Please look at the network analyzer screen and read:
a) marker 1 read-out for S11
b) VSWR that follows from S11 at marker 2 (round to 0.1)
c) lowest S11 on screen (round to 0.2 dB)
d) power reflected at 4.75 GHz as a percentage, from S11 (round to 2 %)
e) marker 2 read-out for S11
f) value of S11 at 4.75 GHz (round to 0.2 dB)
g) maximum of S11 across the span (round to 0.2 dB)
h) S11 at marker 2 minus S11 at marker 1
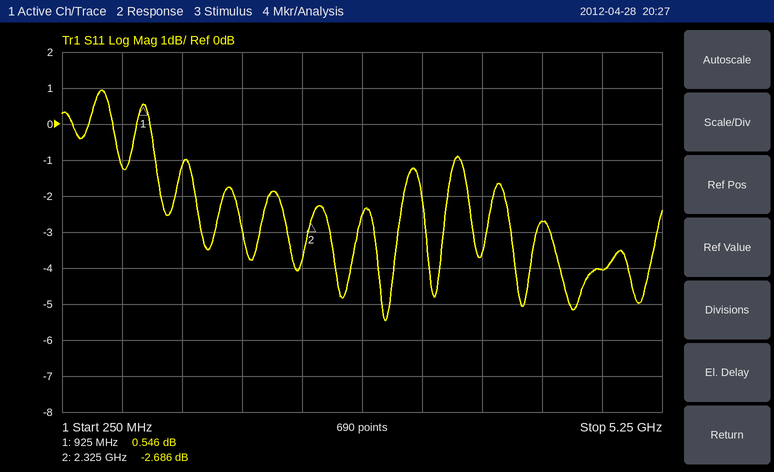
0.546 dB
6.5
-5.4 dB
40 %
-2.686 dB
-4.0 dB
1.0 dB
-3.232 dB
